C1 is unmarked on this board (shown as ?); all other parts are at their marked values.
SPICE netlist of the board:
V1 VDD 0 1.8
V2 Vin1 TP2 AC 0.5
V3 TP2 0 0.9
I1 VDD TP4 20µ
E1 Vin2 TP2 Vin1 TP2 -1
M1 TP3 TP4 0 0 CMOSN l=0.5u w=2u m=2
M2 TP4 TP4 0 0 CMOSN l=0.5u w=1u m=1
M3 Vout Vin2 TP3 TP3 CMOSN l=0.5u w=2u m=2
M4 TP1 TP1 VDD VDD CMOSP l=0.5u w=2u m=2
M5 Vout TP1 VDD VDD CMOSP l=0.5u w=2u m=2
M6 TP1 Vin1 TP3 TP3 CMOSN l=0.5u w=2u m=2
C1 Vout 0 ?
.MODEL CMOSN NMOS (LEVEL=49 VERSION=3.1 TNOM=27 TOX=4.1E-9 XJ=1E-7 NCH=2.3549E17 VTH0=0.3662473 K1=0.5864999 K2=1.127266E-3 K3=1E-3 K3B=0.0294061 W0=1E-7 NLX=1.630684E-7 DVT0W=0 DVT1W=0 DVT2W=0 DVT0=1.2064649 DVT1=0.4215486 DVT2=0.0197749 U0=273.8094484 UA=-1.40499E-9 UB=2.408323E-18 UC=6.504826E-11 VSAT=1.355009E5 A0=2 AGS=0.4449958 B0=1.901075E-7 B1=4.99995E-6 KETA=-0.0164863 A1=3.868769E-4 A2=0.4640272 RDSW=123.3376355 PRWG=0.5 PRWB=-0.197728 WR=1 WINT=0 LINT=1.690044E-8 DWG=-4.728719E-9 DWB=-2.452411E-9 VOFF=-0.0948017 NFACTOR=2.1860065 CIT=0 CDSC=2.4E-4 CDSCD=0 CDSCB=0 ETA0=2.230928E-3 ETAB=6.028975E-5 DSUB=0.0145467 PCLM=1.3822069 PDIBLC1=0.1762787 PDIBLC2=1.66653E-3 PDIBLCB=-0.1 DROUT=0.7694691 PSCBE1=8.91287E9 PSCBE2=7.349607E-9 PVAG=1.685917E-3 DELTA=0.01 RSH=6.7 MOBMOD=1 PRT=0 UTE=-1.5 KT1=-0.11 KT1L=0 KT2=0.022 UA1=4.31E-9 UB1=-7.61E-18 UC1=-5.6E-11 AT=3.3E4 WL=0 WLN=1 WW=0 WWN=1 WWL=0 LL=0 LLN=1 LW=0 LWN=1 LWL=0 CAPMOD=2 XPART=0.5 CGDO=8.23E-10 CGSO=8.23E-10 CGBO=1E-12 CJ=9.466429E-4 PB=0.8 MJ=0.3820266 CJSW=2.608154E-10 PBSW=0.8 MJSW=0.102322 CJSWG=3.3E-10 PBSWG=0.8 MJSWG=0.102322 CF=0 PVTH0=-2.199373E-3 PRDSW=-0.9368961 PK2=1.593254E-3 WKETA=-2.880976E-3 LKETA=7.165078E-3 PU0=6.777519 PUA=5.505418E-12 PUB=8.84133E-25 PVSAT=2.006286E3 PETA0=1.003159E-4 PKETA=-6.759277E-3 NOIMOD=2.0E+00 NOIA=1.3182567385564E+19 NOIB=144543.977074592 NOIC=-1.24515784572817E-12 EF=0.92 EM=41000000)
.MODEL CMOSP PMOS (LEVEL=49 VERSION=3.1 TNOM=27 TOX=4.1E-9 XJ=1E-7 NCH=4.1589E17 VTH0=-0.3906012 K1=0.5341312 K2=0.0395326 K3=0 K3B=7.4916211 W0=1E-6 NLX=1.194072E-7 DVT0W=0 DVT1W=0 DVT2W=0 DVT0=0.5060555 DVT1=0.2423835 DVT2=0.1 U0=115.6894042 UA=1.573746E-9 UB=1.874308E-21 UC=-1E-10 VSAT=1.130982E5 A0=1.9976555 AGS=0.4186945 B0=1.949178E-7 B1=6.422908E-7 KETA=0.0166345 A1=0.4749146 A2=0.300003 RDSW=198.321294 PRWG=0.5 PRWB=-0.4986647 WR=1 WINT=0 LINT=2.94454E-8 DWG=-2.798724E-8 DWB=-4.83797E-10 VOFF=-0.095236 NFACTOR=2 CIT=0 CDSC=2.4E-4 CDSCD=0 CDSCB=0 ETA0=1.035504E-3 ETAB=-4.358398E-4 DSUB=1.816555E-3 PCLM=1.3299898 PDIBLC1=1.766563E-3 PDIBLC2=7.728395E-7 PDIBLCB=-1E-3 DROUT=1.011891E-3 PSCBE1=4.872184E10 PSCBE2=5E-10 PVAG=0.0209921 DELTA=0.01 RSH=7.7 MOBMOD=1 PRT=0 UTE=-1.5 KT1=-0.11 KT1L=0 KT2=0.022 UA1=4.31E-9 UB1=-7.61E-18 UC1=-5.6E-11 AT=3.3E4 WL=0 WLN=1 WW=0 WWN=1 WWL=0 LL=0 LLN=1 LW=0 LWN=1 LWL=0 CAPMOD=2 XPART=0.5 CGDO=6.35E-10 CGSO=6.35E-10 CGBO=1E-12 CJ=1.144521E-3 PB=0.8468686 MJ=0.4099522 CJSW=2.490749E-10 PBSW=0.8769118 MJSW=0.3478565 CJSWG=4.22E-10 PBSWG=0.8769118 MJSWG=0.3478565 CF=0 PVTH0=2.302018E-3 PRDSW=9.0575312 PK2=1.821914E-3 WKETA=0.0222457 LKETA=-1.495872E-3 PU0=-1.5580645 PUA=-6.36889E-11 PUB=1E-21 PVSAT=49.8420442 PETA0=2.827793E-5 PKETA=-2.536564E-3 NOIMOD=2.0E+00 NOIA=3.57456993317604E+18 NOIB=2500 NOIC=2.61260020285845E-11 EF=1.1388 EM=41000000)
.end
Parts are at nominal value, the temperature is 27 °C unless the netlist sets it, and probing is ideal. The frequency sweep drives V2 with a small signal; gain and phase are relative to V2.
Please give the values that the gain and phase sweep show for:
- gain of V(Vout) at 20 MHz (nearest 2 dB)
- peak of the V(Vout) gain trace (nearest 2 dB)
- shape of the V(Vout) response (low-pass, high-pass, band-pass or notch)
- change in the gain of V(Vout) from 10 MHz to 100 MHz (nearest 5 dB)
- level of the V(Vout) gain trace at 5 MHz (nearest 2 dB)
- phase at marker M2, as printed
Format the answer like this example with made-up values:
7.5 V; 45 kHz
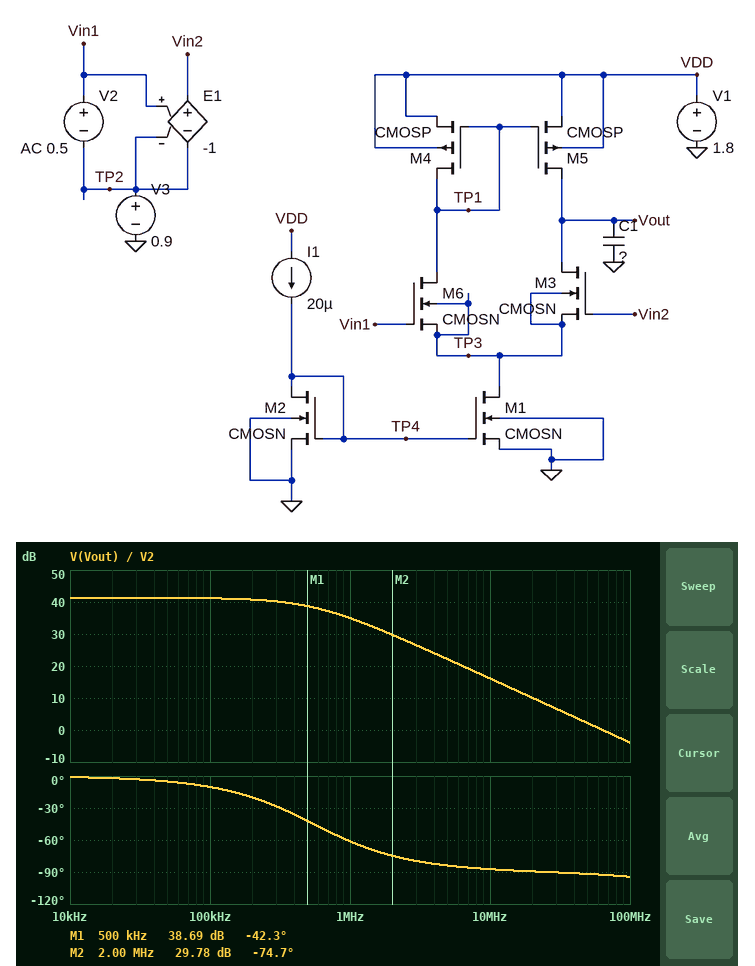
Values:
10 dB; 42 dB; low-pass; -20 dB; 22 dB; -74.7 deg
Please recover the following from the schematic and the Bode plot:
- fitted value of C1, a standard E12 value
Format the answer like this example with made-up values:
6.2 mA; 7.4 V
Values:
1.8 pF
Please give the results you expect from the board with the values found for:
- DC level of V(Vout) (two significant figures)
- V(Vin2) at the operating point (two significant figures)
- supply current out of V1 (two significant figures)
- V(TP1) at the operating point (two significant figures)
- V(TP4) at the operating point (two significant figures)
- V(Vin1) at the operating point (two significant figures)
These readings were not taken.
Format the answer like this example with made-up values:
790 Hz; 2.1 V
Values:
980 mV; 900 mV; 91 µA; 980 mV; 720 mV; 900 mV
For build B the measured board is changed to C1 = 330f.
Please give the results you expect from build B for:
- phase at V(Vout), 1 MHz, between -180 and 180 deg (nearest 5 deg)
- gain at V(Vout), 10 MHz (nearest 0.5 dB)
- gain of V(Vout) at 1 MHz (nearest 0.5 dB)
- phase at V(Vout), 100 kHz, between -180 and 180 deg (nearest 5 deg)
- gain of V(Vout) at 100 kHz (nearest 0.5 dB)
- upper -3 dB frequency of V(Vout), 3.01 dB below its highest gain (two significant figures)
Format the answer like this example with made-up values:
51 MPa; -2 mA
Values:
-20 deg; 30.5 dB; 41.0 dB; 0 deg; 41.5 dB; 2.9 MHz
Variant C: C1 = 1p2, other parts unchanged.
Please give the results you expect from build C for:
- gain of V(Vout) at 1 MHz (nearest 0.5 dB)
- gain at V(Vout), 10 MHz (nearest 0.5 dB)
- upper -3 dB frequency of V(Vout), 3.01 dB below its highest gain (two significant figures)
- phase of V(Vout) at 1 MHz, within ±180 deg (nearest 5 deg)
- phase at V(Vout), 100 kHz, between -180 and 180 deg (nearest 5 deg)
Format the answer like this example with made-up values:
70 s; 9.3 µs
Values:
37.5 dB; 19.5 dB; 820 kHz; -50 deg; -5 deg
